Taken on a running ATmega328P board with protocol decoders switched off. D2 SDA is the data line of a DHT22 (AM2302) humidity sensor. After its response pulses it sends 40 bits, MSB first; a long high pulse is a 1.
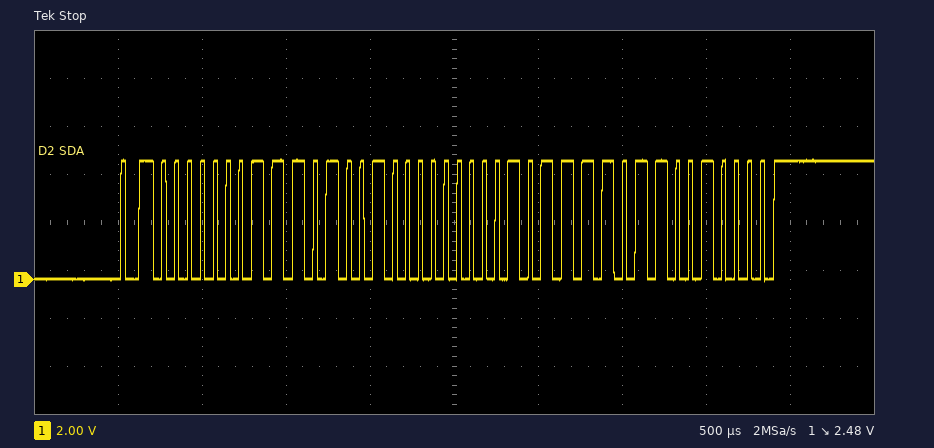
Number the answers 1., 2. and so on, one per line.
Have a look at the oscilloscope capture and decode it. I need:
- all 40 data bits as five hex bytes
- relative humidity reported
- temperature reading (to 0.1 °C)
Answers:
1. 01 D2 00 BD 90
2. 46.6 %
3. 18.9 °C
